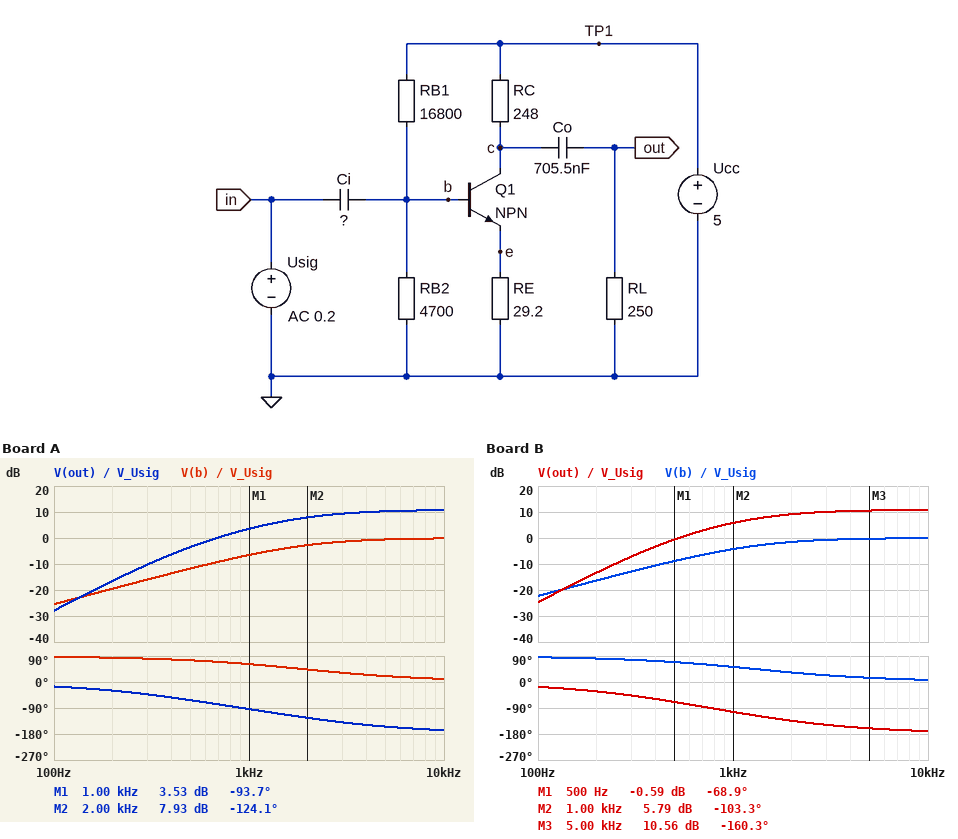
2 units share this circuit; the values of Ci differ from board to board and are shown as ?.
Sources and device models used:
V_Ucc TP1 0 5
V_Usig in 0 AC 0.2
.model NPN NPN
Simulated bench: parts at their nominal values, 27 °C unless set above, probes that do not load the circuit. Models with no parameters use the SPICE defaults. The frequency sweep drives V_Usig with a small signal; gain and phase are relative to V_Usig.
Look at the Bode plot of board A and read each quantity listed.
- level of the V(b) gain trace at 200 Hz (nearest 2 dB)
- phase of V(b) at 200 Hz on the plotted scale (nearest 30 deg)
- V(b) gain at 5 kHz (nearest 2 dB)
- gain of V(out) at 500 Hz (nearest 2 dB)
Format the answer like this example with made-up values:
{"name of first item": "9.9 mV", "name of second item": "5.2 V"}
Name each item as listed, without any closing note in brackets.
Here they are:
{"level of the V(b) gain trace at 200 Hz": "-20 dB", "phase of V(b) at 200 Hz on the plotted scale": "90 deg", "V(b) gain at 5 kHz": "0 dB", "gain of V(out) at 500 Hz": "-4 dB"}
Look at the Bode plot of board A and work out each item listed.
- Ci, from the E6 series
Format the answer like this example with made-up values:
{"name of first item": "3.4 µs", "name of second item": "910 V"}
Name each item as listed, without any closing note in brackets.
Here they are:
{"Ci, from the E6 series": "47 nF"}
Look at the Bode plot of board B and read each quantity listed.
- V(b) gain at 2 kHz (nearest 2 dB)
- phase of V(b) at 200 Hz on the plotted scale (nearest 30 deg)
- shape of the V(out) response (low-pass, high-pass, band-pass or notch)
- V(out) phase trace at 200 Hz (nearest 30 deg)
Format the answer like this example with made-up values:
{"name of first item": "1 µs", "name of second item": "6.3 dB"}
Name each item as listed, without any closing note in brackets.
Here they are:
{"V(b) gain at 2 kHz": "-2 dB", "phase of V(b) at 200 Hz on the plotted scale": "90 deg", "shape of the V(out) response": "high-pass", "V(out) phase trace at 200 Hz": "-30 deg"}
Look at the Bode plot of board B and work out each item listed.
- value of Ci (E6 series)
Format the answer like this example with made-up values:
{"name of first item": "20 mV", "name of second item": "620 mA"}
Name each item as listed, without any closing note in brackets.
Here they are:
{"value of Ci": "68 nF"}
